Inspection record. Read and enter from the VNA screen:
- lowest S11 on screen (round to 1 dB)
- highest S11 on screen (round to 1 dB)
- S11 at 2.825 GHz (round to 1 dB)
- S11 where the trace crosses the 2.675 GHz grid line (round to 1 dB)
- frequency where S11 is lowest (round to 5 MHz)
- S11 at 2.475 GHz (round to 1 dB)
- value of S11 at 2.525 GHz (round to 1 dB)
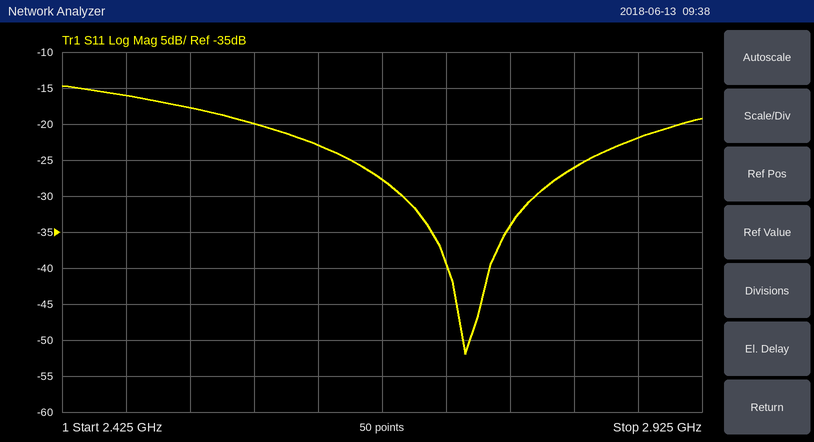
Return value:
-52 dB
-15 dB
-26 dB
-28 dB
2.740 GHz
-16 dB
-18 dB
